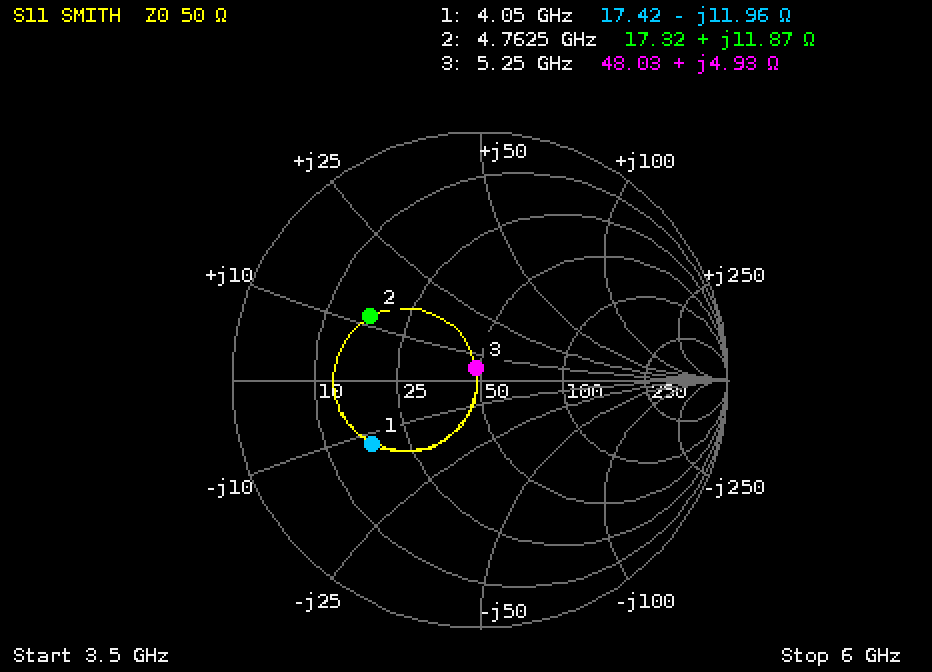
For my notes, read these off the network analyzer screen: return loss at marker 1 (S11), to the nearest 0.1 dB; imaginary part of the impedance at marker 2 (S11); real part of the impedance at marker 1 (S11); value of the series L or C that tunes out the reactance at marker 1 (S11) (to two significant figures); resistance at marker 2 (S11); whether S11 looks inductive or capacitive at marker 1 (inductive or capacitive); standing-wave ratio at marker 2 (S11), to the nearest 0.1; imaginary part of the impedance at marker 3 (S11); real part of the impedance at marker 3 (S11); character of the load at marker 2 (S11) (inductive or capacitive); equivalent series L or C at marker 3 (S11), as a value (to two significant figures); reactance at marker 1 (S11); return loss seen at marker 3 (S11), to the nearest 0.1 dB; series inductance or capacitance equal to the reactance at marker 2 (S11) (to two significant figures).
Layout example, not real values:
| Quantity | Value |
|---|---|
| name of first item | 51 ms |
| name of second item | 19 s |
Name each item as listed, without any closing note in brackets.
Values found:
| Quantity | Value |
|---|---|
| return loss at marker 1 (S11), to the nearest 0.1 dB | 5.9 dB |
| imaginary part of the impedance at marker 2 | +11.87 Ω |
| real part of the impedance at marker 1 | 17.42 Ω |
| value of the series L or C that tunes out the reactance at marker 1 (S11) | 470 pH |
| resistance at marker 2 | 17.32 Ω |
| whether S11 looks inductive or capacitive at marker 1 | capacitive |
| standing-wave ratio at marker 2 (S11), to the nearest 0.1 | 3.1 |
| imaginary part of the impedance at marker 3 | +4.93 Ω |
| real part of the impedance at marker 3 | 48.03 Ω |
| character of the load at marker 2 (S11) | inductive |
| equivalent series L or C at marker 3 (S11), as a value | 150 pH |
| reactance at marker 1 | -11.96 Ω |
| return loss seen at marker 3 (S11), to the nearest 0.1 dB | 25.3 dB |
| series inductance or capacitance equal to the reactance at marker 2 (S11) | 400 pH |
